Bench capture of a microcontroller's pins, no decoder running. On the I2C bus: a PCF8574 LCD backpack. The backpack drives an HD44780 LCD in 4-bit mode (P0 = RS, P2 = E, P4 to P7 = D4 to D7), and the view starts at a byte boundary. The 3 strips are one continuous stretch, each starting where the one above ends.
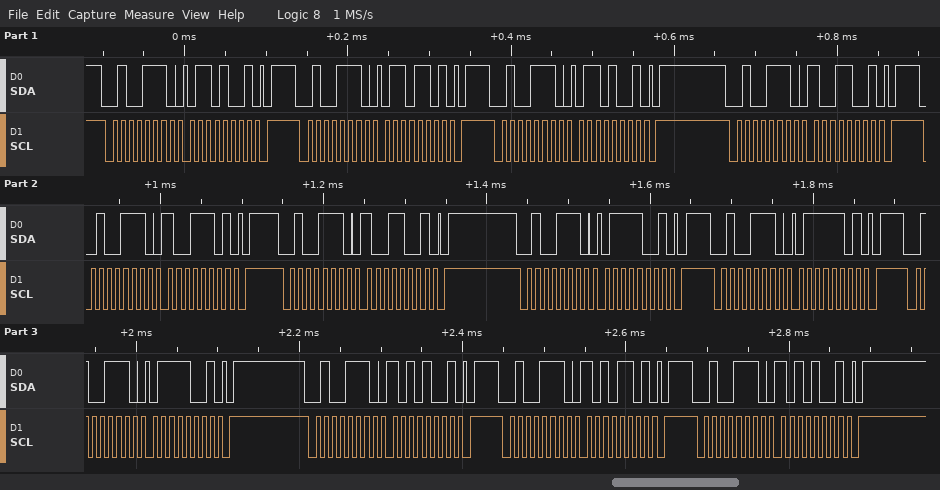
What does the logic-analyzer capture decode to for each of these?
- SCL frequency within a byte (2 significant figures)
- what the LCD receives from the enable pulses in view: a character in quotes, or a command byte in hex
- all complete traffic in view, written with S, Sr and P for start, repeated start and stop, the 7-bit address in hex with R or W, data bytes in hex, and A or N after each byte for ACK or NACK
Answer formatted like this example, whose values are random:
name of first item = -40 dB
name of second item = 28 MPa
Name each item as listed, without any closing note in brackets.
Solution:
SCL frequency within a byte = 100 kHz
what the LCD receives from the enable pulses in view: a character in quotes, or a command byte in hex = 'i' 'z'
all complete traffic in view, written with S, Sr and P for start, repeated start and stop, the 7-bit address in hex with R or W, data bytes in hex, and A or N after each byte for ACK or NACK = S 27W A 69 A P S 27W A 6D A P S 27W A 69 A P S 27W A 99 A P S 27W A 9D A P S 27W A 99 A P S 27W A 79 A P S 27W A 7D A P S 27W A 79 A P S 27W A A9 A P S 27W A AD A P S 27W A A9 A P
